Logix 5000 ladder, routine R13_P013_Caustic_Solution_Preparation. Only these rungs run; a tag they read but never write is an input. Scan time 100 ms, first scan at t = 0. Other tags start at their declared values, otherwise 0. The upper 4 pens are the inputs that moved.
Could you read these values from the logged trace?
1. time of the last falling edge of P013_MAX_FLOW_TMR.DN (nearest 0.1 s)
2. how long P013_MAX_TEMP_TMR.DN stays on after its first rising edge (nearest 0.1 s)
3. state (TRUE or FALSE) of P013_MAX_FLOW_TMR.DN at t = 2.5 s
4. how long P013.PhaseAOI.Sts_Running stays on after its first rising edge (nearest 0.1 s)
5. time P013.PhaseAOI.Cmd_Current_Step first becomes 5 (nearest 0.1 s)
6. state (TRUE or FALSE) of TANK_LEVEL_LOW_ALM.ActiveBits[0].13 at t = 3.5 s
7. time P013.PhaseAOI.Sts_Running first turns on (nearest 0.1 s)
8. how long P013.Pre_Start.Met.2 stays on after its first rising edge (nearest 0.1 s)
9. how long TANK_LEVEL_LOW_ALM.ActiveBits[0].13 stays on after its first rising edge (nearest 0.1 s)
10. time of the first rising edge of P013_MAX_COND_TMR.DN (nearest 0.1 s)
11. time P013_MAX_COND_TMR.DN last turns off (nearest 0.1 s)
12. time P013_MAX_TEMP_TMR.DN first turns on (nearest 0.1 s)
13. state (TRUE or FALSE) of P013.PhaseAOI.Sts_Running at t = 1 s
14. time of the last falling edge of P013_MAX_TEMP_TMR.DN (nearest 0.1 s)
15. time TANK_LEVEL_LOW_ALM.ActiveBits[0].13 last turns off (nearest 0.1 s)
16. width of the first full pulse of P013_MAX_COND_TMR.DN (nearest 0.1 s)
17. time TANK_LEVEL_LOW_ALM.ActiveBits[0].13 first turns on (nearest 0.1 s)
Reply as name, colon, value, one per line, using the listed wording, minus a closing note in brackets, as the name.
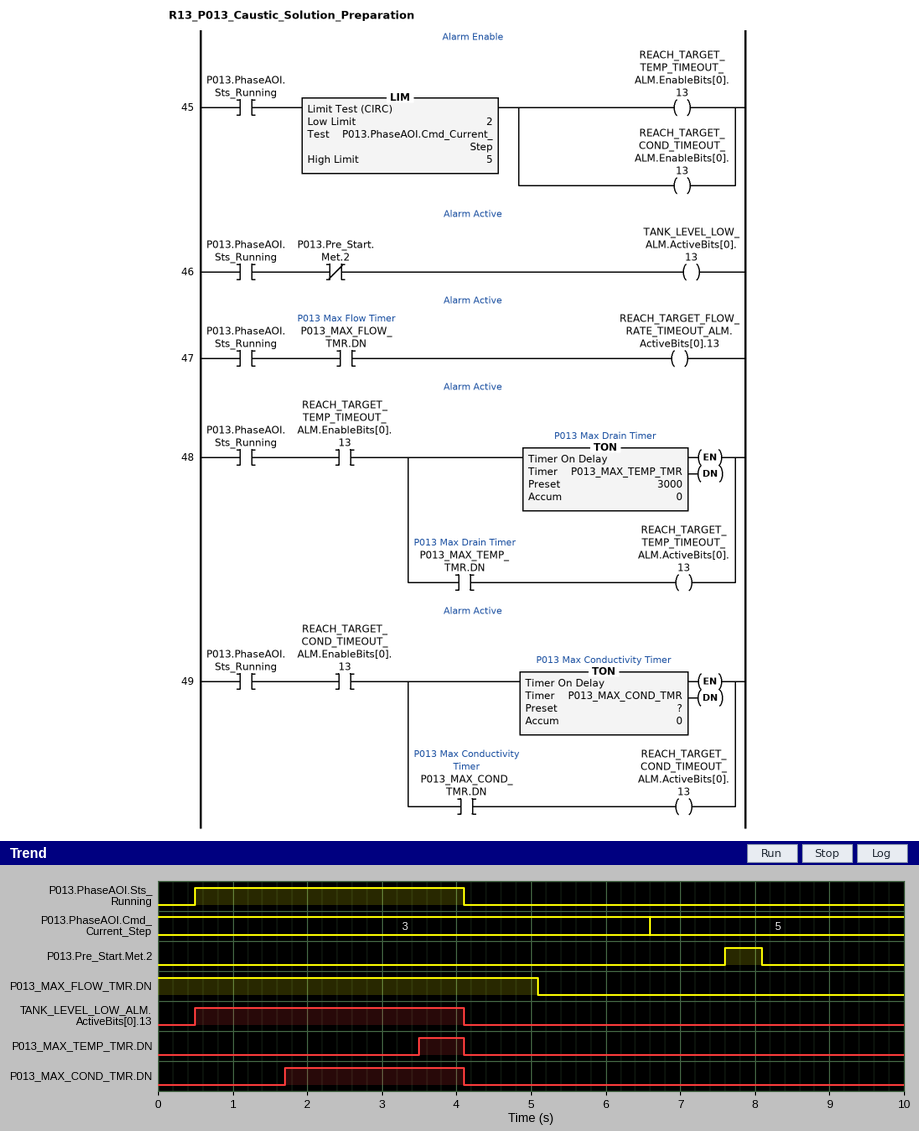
time of the last falling edge of P013_MAX_FLOW_TMR.DN: 5.1 s
how long P013_MAX_TEMP_TMR.DN stays on after its first rising edge: 0.6 s
state (TRUE or FALSE) of P013_MAX_FLOW_TMR.DN at t = 2.5 s: TRUE
how long P013.PhaseAOI.Sts_Running stays on after its first rising edge: 3.6 s
time P013.PhaseAOI.Cmd_Current_Step first becomes 5: 6.6 s
state (TRUE or FALSE) of TANK_LEVEL_LOW_ALM.ActiveBits[0].13 at t = 3.5 s: TRUE
time P013.PhaseAOI.Sts_Running first turns on: 0.5 s
how long P013.Pre_Start.Met.2 stays on after its first rising edge: 0.5 s
how long TANK_LEVEL_LOW_ALM.ActiveBits[0].13 stays on after its first rising edge: 3.6 s
time of the first rising edge of P013_MAX_COND_TMR.DN: 1.7 s
time P013_MAX_COND_TMR.DN last turns off: 4.1 s
time P013_MAX_TEMP_TMR.DN first turns on: 3.5 s
state (TRUE or FALSE) of P013.PhaseAOI.Sts_Running at t = 1 s: TRUE
time of the last falling edge of P013_MAX_TEMP_TMR.DN: 4.1 s
time TANK_LEVEL_LOW_ALM.ActiveBits[0].13 last turns off: 4.1 s
width of the first full pulse of P013_MAX_COND_TMR.DN: 2.4 s
time TANK_LEVEL_LOW_ALM.ActiveBits[0].13 first turns on: 0.5 s
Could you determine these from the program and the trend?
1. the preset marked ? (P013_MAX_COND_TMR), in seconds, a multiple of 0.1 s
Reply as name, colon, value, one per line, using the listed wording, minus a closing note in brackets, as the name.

the preset marked ? (P013_MAX_COND_TMR), in seconds, a multiple of 0.1 s: 1.2 s
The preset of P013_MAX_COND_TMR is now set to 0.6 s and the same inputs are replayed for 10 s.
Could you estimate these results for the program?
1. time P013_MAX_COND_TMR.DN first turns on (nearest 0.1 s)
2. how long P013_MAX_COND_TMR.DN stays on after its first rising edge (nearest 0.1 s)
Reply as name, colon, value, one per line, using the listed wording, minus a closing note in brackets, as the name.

time P013_MAX_COND_TMR.DN first turns on: 1.1 s
how long P013_MAX_COND_TMR.DN stays on after its first rising edge: 3.0 s
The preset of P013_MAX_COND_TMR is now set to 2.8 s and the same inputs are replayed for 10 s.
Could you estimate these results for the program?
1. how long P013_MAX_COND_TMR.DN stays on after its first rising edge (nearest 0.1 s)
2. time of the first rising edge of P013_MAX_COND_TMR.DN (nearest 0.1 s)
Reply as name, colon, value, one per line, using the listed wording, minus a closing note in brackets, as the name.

how long P013_MAX_COND_TMR.DN stays on after its first rising edge: 0.8 s
time of the first rising edge of P013_MAX_COND_TMR.DN: 3.3 s
